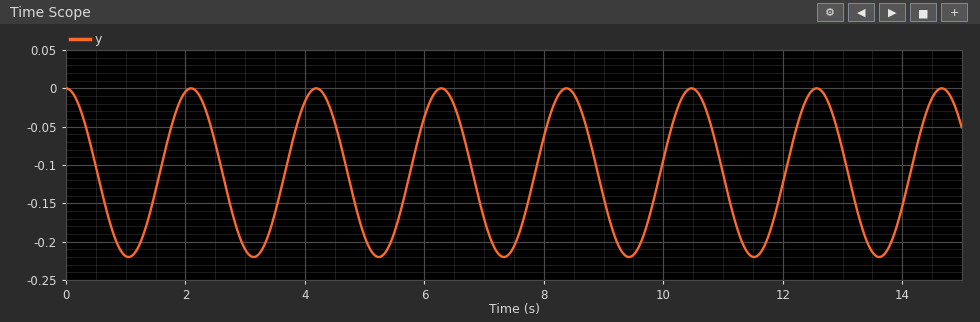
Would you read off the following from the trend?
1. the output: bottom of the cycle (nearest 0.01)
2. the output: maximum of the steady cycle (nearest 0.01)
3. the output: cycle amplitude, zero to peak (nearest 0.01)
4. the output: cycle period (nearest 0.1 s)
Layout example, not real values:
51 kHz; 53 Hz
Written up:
-0.22; 0.00; 0.11; 2.1 s
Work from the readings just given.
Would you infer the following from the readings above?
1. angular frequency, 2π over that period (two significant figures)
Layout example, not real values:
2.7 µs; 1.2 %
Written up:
3.0 rad/s
